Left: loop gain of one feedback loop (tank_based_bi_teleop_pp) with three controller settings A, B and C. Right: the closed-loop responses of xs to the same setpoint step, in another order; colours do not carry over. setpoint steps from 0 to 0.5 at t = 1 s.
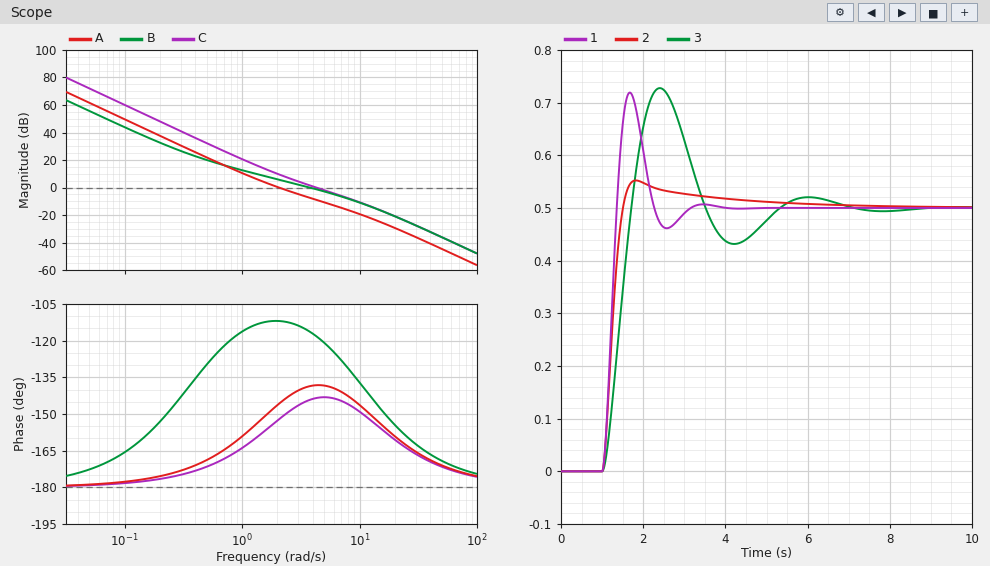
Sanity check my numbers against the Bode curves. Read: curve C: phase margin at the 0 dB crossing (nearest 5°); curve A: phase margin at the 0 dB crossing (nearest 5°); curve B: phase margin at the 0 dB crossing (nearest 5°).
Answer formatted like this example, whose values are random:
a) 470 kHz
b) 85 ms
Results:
a) 35°
b) 35°
c) 65°
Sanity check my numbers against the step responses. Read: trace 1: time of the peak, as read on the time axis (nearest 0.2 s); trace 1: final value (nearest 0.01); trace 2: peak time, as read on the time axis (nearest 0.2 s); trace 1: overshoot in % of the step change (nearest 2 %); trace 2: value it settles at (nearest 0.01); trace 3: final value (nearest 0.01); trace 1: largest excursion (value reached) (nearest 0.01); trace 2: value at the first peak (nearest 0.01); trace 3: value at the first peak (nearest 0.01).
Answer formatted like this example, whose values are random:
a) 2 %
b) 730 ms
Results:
a) 1.6 s
b) 0.50
c) 1.8 s
d) 44 %
e) 0.50
f) 0.50
g) 0.72
h) 0.55
i) 0.73
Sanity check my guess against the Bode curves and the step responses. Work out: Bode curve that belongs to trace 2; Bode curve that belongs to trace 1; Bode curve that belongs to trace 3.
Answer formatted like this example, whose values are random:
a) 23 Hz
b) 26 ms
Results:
a) B
b) C
c) A
